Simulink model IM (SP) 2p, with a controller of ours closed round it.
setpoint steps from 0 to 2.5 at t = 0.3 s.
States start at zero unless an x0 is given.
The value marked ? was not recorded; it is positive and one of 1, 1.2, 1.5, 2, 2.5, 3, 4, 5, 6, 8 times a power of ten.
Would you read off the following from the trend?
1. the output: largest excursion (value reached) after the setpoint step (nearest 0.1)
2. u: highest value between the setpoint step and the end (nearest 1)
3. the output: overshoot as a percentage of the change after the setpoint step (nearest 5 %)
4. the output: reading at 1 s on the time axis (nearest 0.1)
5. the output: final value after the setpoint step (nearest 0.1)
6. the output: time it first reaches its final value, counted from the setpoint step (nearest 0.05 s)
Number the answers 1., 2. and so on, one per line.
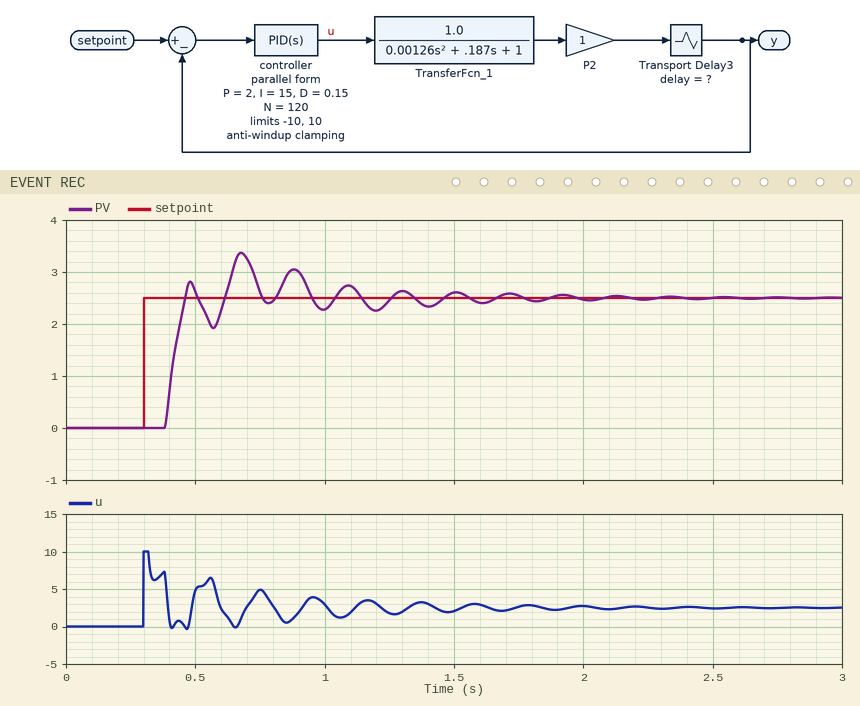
1. 3.4
2. 10
3. 35 %
4. 2.3
5. 2.5
6. 0.15 s
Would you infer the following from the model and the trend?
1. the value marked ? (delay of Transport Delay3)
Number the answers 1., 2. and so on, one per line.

1. 0.08
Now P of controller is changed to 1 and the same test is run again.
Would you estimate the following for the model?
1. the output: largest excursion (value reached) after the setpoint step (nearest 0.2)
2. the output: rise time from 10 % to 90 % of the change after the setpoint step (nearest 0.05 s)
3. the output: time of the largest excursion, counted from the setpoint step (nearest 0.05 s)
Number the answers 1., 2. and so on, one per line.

1. 3.4
2. 0.20 s
3. 0.55 s
